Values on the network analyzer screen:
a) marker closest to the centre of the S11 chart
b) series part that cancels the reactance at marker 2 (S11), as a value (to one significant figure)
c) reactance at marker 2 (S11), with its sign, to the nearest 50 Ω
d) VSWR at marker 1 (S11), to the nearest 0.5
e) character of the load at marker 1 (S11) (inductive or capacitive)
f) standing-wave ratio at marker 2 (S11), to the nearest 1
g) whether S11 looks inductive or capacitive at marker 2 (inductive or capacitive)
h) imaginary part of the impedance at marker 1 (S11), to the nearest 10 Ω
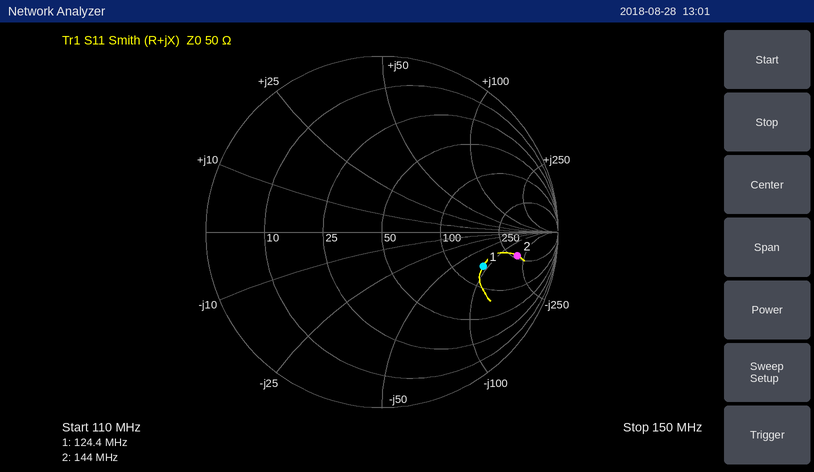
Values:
marker 1
200 nH
-200 Ω
4.0
capacitive
8
capacitive
-90 Ω
